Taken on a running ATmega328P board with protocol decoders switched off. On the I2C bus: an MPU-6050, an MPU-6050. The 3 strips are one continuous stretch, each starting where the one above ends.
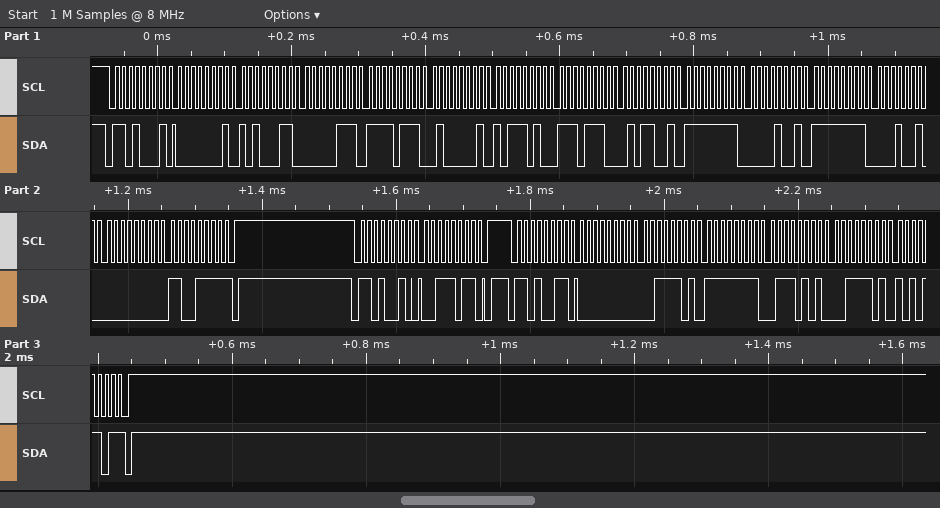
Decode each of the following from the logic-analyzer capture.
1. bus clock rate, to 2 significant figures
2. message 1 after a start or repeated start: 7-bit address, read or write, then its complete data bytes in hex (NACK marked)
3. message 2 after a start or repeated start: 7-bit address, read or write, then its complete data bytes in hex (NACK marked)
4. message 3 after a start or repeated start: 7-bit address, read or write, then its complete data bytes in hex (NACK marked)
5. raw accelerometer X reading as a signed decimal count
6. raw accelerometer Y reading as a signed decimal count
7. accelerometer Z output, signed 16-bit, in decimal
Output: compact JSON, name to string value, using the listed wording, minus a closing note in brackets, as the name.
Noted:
{"bus clock rate, to 2 significant figures": "100 kHz", "message 1 after a start or repeated start: 7-bit address, read or write, then its complete data bytes in hex": "0x68 read: 01 A3 07 F7 41 BA EE 59 FF 09 FF 12 00 CF NACK", "message 2 after a start or repeated start: 7-bit address, read or write, then its complete data bytes in hex": "0x69 write: 3B", "message 3 after a start or repeated start: 7-bit address, read or write, then its complete data bytes in hex": "0x69 read: 00 3D FF 75 3D AD NACK", "raw accelerometer X reading as a signed decimal count": "61", "raw accelerometer Y reading as a signed decimal count": "-139", "accelerometer Z output, signed 16-bit, in decimal": "15789"}
